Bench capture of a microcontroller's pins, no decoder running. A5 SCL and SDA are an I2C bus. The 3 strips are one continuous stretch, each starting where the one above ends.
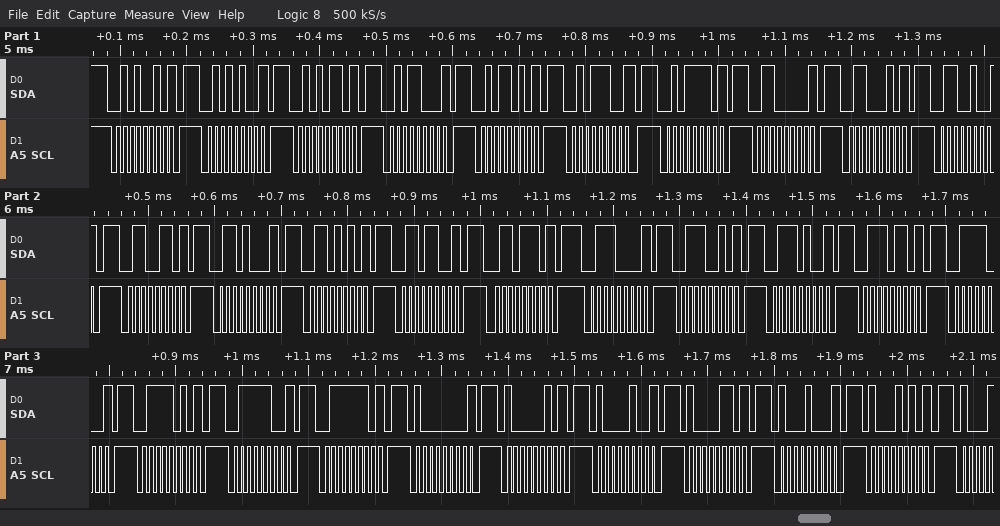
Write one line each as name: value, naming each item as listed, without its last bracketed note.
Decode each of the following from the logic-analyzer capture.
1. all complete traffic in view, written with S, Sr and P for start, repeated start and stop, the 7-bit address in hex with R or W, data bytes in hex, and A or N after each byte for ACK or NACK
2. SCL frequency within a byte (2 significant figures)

all complete traffic in view, written with S, Sr and P for start, repeated start and stop, the 7-bit address in hex with R or W, data bytes in hex, and A or N after each byte for ACK or NACK: S 29W N P S 2AW N P S 2BW N P S 2CW N P S 2DW N P S 2EW N P S 2FW N P S 30W N P S 31W N P S 32W N P S 33W N P S 34W N P S 35W N P S 36W N P S 37W N P S 38W N P S 39W N P S 3AW N P S 3BW N P S 3CW N P S 3DW N P S 3EW N P S 3FW N P S 40W N P S 41W N P S 42W N P S 43W N P S 44W N P S 45W N P
SCL frequency within a byte: 100 kHz
